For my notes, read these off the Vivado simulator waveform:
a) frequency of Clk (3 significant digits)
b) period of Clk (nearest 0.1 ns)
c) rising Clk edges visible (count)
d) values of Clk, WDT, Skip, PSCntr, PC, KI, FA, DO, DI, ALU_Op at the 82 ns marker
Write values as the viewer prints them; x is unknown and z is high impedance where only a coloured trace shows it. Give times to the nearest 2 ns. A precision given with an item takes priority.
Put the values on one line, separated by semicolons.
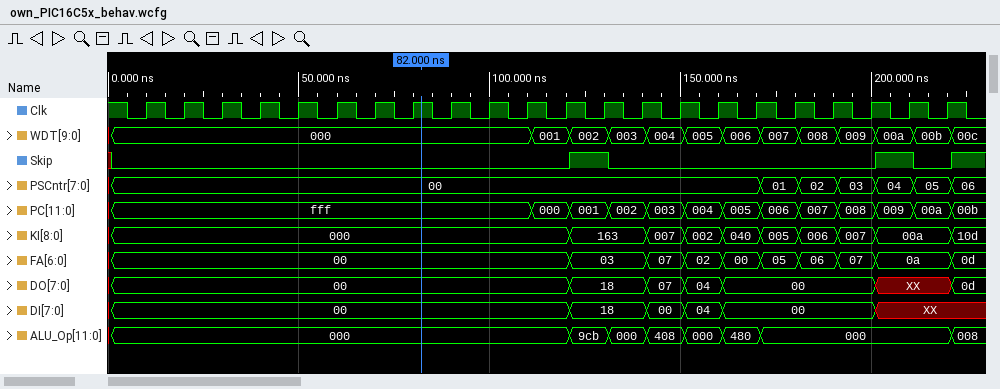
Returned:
100 MHz; 10 ns; 22; Clk=1, WDT=000, Skip=0, PSCntr=00, PC=fff, KI=000, FA=00, DO=00, DI=00, ALU_Op=000
